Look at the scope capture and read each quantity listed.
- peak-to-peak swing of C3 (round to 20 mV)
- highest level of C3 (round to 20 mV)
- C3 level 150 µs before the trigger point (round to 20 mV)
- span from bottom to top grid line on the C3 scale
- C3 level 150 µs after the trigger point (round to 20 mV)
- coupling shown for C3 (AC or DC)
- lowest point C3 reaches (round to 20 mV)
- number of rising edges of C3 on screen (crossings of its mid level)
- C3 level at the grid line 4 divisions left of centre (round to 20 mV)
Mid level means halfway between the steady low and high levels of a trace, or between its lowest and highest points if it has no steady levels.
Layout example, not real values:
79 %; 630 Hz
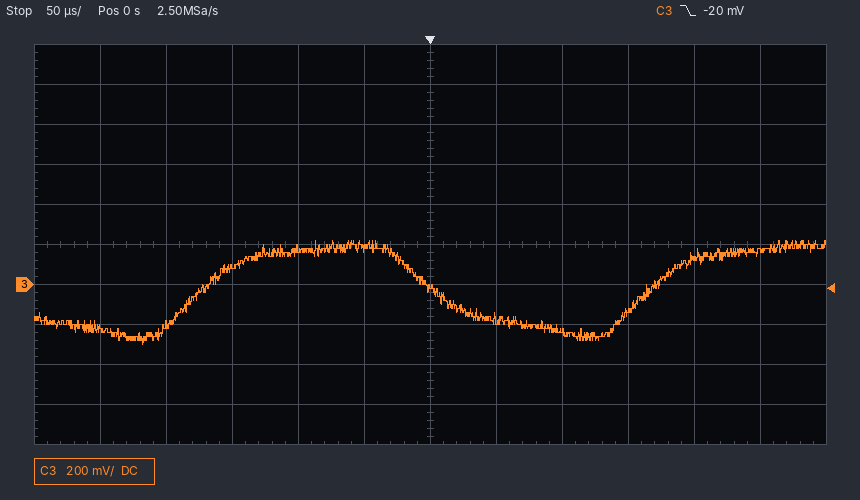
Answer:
520 mV; 220 mV; 80 mV; 2 V; -140 mV; DC; -300 mV; 2; -200 mV
